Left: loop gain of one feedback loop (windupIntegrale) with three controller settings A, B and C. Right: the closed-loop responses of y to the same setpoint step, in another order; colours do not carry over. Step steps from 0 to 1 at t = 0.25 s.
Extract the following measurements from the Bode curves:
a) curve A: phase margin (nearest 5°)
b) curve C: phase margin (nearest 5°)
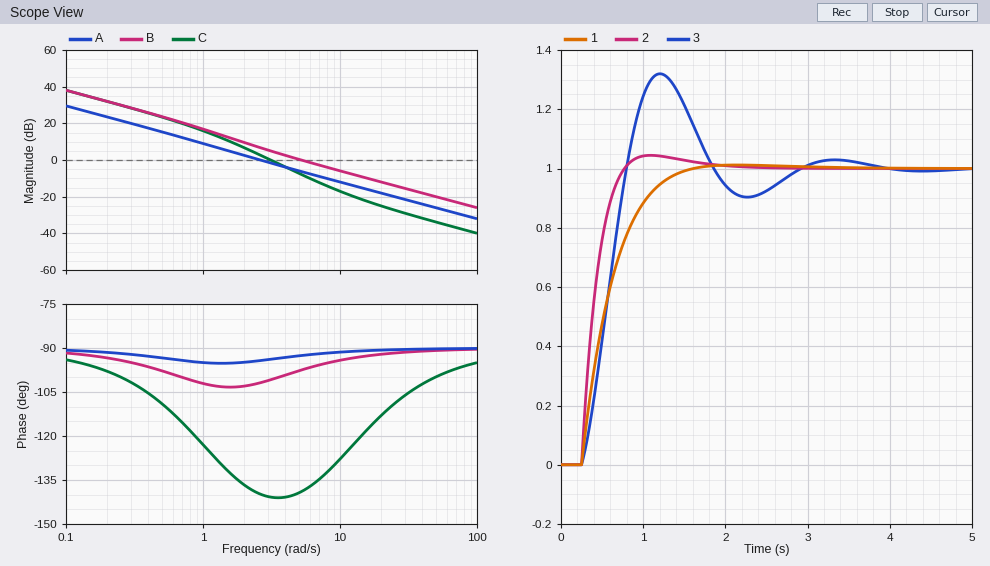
85°
40°
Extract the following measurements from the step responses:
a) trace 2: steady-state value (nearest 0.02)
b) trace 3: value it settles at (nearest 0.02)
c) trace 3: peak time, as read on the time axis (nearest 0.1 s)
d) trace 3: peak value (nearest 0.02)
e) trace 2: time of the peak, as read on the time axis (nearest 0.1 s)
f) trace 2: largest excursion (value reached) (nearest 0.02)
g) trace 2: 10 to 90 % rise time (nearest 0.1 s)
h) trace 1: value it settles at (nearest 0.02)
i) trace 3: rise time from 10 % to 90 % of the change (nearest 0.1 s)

1.00
1.00
1.2 s
1.32
1.1 s
1.04
0.3 s
1.00
0.4 s
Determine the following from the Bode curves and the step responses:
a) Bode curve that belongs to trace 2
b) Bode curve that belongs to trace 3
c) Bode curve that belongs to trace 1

B
C
A
